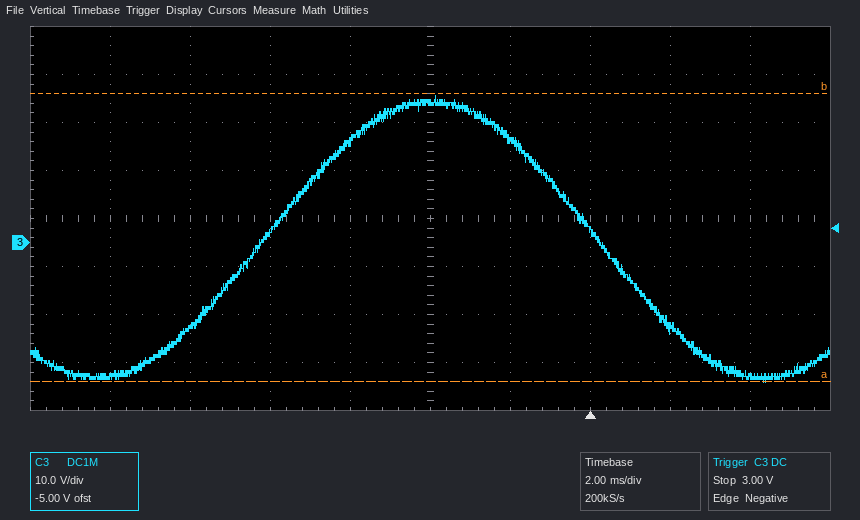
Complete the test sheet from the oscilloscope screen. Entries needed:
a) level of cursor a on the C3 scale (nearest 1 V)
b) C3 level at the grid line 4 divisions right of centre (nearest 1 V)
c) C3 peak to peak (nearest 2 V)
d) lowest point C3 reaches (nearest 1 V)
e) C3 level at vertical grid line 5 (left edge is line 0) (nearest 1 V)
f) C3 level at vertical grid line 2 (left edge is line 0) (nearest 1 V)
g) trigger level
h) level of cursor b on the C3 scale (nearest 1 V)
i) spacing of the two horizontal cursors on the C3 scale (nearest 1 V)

-29 V
-28 V
60 V
-29 V
29 V
-18 V
3.00 V
31 V
60 V
